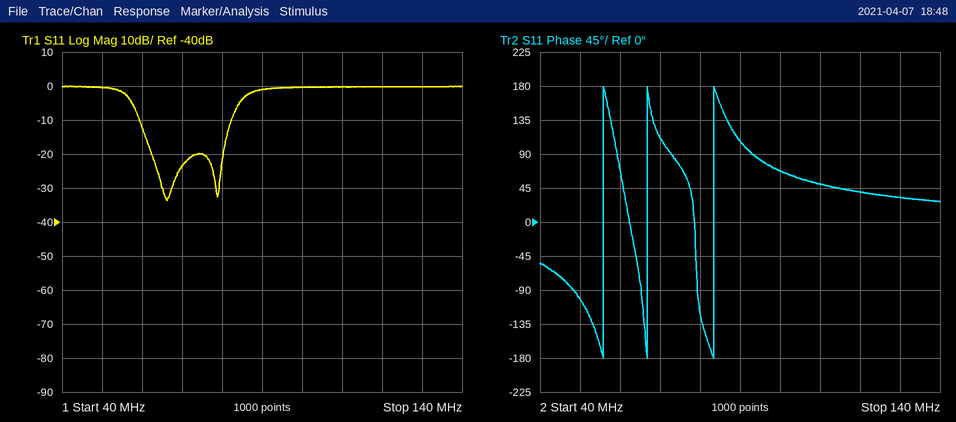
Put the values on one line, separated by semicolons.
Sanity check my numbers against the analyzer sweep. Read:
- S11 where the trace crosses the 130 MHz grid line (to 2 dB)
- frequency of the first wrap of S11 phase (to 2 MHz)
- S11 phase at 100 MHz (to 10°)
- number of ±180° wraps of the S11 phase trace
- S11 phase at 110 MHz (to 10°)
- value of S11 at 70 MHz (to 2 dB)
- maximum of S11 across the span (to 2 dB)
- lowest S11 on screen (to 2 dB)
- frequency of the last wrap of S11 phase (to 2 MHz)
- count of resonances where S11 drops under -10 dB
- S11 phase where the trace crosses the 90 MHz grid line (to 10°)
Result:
0 dB; 56 MHz; 70°; 3; 50°; -24 dB; 0 dB; -34 dB; 84 MHz; 2; 110°
